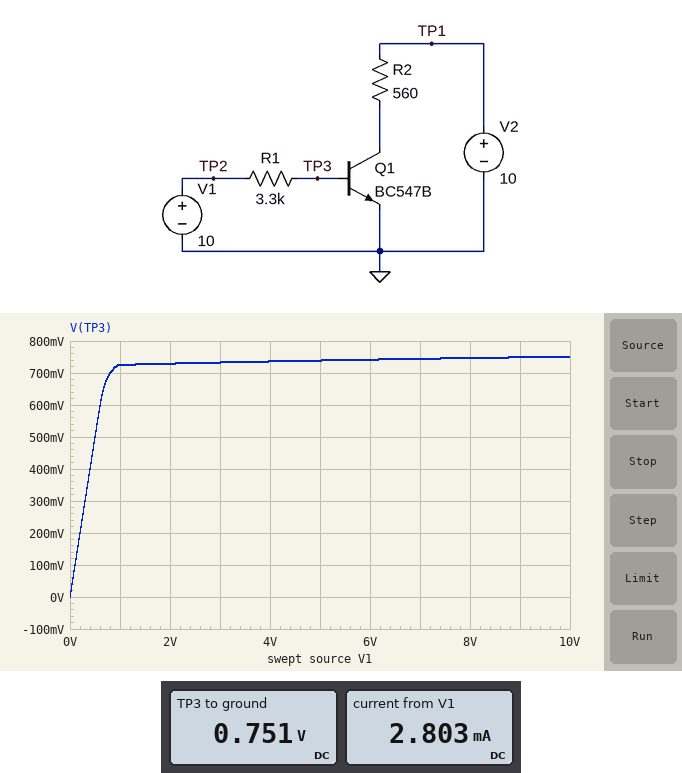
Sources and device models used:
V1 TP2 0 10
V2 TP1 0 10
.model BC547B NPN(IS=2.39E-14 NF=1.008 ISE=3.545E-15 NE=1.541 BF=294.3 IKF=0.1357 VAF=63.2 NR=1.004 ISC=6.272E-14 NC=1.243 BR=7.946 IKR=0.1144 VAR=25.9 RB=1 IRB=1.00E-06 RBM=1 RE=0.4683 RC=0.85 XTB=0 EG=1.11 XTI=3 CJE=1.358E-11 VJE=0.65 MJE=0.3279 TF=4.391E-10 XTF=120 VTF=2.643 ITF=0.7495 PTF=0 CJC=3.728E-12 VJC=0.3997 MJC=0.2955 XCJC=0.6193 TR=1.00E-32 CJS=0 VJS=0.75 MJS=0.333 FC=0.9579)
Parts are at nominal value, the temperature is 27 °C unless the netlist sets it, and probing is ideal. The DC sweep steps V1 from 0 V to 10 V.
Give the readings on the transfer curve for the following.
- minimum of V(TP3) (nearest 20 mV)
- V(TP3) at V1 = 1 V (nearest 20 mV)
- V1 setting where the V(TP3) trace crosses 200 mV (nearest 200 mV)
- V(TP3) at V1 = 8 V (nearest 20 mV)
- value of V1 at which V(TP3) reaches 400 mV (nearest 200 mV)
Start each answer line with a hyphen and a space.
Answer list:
- 0 V
- 720 mV
- 200 mV
- 740 mV
- 400 mV
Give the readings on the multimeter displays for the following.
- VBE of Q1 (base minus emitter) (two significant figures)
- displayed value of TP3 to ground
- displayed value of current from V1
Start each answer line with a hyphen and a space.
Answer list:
- 750 mV
- 0.751 V
- 2.803 mA
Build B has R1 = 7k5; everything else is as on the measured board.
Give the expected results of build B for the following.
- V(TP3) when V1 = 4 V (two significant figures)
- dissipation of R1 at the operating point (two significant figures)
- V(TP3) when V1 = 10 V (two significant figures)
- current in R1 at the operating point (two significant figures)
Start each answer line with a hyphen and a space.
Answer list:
- 730 mV
- 11 mW
- 740 mV
- 1.2 mA
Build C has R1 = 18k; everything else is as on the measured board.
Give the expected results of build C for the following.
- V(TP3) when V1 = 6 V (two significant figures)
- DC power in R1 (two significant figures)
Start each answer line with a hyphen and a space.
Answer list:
- 730 mV
- 4.8 mW
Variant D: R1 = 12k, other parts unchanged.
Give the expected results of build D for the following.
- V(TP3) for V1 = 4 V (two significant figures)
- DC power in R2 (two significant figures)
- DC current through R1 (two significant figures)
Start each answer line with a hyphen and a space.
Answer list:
- 730 mV
- 180 mW
- 770 µA
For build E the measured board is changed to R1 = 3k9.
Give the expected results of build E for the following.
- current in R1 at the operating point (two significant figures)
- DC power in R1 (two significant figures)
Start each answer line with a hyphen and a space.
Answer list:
- 2.4 mA
- 22 mW
